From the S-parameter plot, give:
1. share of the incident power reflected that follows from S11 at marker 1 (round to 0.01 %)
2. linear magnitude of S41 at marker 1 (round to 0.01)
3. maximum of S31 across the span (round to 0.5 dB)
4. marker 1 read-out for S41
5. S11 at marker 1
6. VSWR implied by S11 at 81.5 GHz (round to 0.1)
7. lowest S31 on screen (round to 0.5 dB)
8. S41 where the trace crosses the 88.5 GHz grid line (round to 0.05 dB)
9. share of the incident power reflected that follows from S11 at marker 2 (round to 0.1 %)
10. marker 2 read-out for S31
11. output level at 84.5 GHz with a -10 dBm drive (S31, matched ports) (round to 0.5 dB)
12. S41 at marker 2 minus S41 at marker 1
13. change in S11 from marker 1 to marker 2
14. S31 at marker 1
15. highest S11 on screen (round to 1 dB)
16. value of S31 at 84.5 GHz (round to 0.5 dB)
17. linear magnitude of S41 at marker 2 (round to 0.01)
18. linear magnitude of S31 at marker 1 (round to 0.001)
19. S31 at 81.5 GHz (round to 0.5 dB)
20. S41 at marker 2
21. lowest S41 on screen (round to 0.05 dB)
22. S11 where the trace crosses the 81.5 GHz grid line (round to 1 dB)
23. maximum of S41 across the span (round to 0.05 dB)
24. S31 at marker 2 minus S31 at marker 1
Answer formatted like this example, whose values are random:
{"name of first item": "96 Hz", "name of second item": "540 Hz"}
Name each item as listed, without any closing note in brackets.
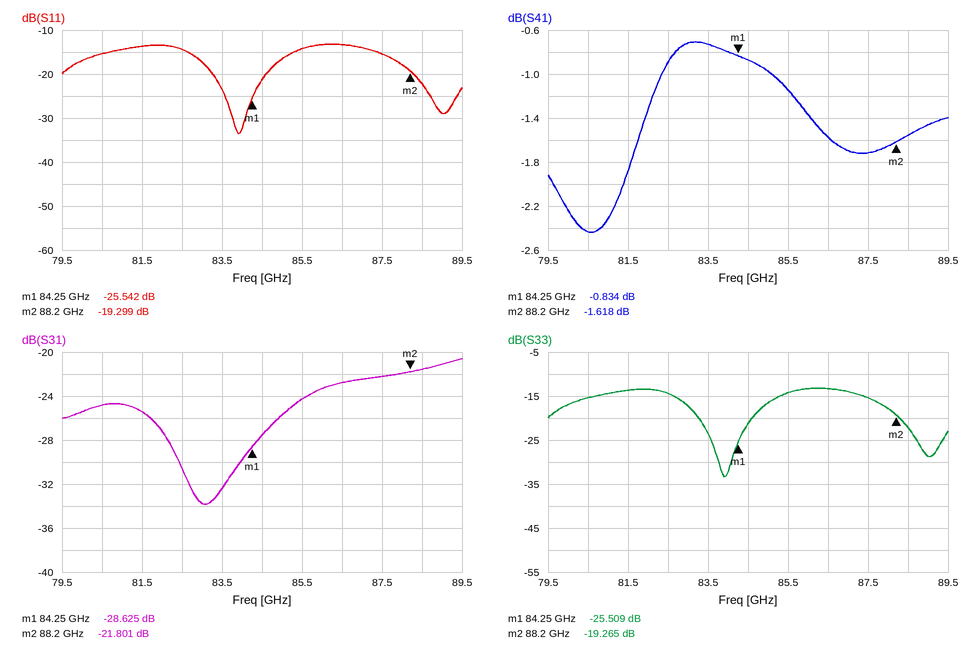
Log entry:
{"share of the incident power reflected that follows from S11 at marker 1": "0.28 %", "linear magnitude of S41 at marker 1": "0.91", "maximum of S31 across the span": "-20.5 dB", "marker 1 read-out for S41": "-0.834 dB", "S11 at marker 1": "-25.542 dB", "VSWR implied by S11 at 81.5 GHz": "1.5", "lowest S31 on screen": "-34.0 dB", "S41 where the trace crosses the 88.5 GHz grid line": "-1.55 dB", "share of the incident power reflected that follows from S11 at marker 2": "1.2 %", "marker 2 read-out for S31": "-21.801 dB", "output level at 84.5 GHz with a -10 dBm drive (S31, matched ports)": "-37.5 dBm", "S41 at marker 2 minus S41 at marker 1": "-0.784 dB", "change in S11 from marker 1 to marker 2": "6.243 dB", "S31 at marker 1": "-28.625 dB", "highest S11 on screen": "-13 dB", "value of S31 at 84.5 GHz": "-27.5 dB", "linear magnitude of S41 at marker 2": "0.83", "linear magnitude of S31 at marker 1": "0.037", "S31 at 81.5 GHz": "-25.5 dB", "S41 at marker 2": "-1.618 dB", "lowest S41 on screen": "-2.45 dB", "S11 where the trace crosses the 81.5 GHz grid line": "-14 dB", "maximum of S41 across the span": "-0.70 dB", "S31 at marker 2 minus S31 at marker 1": "6.824 dB"}
